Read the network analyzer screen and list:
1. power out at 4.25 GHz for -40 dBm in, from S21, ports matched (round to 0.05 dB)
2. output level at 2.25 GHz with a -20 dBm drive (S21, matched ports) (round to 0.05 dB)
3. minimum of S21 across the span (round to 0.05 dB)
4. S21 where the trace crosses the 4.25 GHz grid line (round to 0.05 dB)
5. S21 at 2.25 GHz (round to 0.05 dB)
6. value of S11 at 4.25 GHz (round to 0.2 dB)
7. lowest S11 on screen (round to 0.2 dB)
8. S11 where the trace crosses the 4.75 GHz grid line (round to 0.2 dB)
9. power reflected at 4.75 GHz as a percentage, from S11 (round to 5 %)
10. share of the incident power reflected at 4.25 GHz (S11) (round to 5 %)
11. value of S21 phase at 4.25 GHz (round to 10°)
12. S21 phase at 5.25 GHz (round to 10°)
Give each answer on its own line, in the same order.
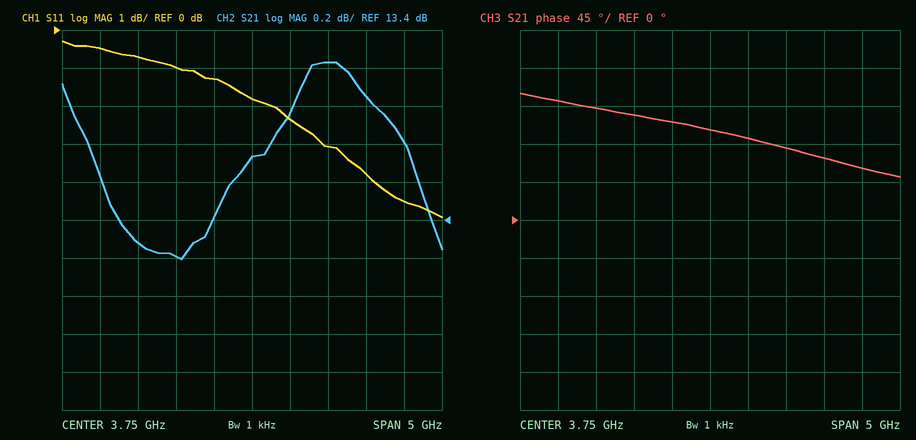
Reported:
-26.05 dBm
-6.70 dBm
13.20 dB
13.95 dB
13.30 dB
-2.4 dB
-5.0 dB
-3.0 dB
50 %
60 %
100°
70°
